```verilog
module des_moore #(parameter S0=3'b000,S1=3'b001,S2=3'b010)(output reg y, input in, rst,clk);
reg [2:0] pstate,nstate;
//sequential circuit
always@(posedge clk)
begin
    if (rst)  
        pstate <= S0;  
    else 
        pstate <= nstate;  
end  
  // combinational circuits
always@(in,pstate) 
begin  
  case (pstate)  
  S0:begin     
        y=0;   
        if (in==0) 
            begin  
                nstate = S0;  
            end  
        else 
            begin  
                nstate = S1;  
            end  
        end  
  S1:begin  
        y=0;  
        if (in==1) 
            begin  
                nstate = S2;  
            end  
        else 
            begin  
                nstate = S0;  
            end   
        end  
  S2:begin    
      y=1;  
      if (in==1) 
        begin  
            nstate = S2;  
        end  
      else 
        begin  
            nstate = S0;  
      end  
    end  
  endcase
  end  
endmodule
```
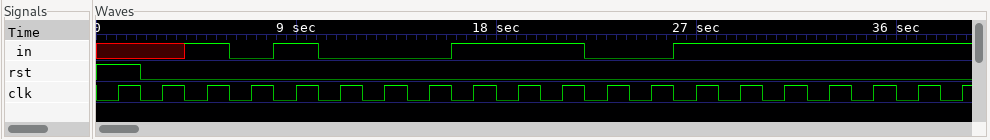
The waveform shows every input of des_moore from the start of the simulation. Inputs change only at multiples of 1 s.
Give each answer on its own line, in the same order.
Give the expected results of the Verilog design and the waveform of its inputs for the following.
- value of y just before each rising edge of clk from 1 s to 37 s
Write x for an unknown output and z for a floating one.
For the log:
x 0 0 1 0 0 0 0 0 0 1 1 0 0 0 1 1 1 1
